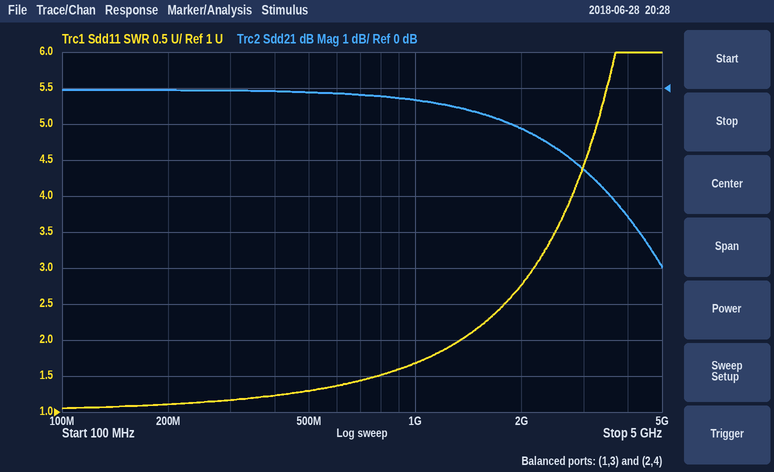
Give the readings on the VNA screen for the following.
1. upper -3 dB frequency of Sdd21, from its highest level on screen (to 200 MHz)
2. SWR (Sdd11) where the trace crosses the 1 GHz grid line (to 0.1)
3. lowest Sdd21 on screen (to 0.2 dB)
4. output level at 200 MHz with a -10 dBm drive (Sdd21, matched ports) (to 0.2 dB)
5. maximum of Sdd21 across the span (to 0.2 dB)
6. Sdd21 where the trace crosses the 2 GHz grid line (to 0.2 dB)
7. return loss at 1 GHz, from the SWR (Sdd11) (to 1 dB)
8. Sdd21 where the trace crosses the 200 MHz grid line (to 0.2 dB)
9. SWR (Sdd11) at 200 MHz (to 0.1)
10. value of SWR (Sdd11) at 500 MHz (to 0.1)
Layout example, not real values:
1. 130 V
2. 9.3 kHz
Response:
1. 3.6 GHz
2. 1.7
3. -5.0 dB
4. -10.0 dBm
5. 0.0 dB
6. -1.2 dB
7. 12 dB
8. 0.0 dB
9. 1.1
10. 1.3
